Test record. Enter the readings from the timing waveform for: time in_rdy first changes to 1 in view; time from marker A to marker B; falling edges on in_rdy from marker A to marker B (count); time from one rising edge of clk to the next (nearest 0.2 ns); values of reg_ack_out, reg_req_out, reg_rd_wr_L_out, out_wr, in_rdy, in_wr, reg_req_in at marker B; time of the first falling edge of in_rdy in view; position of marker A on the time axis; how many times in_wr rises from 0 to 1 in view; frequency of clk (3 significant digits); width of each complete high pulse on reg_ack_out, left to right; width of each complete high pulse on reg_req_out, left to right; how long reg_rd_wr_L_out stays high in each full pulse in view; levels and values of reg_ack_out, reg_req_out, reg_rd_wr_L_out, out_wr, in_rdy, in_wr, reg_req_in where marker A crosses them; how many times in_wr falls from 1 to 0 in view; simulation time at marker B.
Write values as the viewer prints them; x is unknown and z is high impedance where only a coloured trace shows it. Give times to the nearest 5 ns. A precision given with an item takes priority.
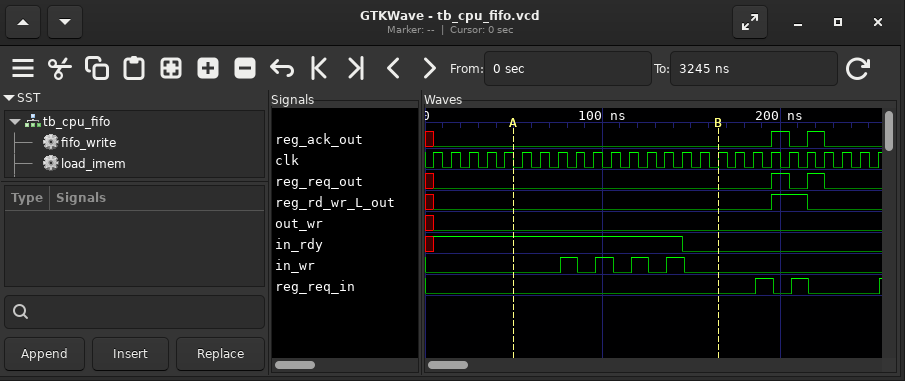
5 ns
115 ns
1
10 ns
reg_ack_out=0, reg_req_out=0, reg_rd_wr_L_out=0, out_wr=0, in_rdy=0, in_wr=0, reg_req_in=0
145 ns
50 ns
4
100 MHz
10 ns, 10 ns
10 ns, 10 ns
20 ns
reg_ack_out=0, reg_req_out=0, reg_rd_wr_L_out=0, out_wr=0, in_rdy=1, in_wr=0, reg_req_in=0
4
165 ns
